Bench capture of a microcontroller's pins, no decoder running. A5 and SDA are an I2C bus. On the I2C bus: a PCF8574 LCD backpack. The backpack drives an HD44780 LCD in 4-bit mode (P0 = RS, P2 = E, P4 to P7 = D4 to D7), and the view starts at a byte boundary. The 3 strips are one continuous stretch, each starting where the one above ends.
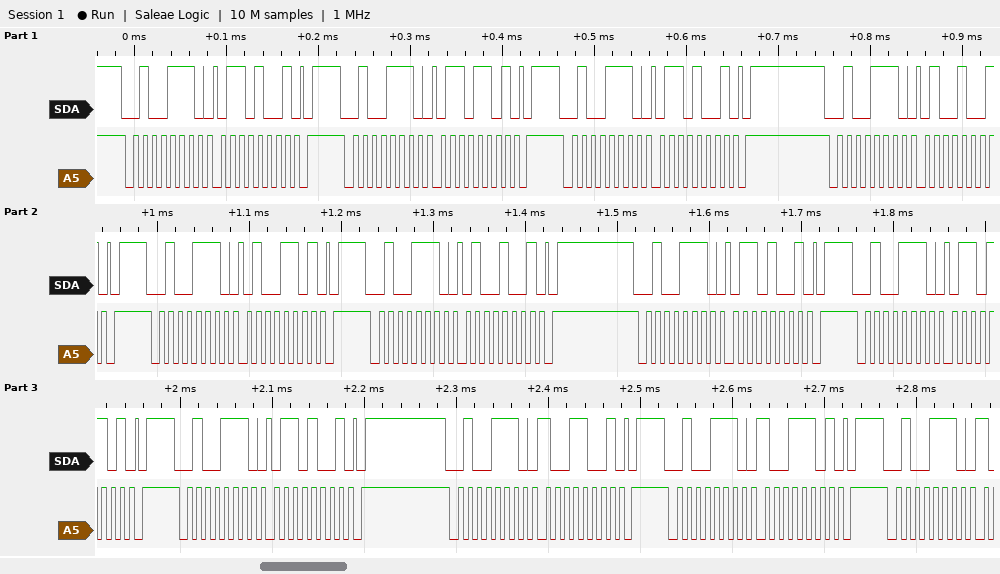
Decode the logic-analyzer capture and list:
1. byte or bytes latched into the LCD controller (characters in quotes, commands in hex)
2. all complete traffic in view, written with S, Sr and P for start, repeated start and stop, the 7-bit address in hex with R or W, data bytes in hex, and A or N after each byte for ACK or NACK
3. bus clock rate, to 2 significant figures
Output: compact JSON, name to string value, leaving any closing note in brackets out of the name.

{"byte or bytes latched into the LCD controller": "'d'", "all complete traffic in view, written with S, Sr and P for start, repeated start and stop, the 7-bit address in hex with R or W, data bytes in hex, and A or N after each byte for ACK or NACK": "S 27W A 69 A P S 27W A 6D A P S 27W A 69 A P S 27W A 49 A P S 27W A 4D A P S 27W A 49 A P S 27W A 69 A P S 27W A 6D A P S 27W A 69 A P S 27W A 99 A P S 27W A 9D A P S 27W A", "bus clock rate, to 2 significant figures": "100 kHz"}
